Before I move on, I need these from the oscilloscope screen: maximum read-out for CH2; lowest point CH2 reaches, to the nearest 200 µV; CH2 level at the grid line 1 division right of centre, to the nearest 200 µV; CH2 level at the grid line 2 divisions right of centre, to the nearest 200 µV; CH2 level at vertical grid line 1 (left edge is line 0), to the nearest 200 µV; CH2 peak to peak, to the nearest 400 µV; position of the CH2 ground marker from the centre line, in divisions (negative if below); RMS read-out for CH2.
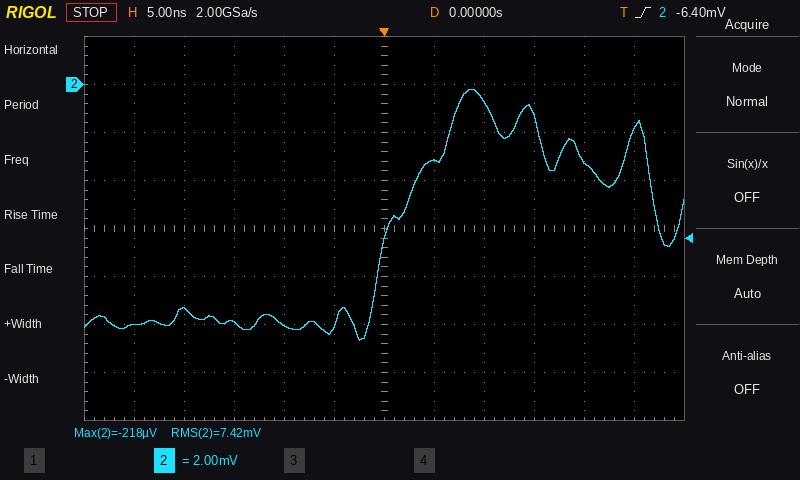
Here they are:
-218 µV
-10.6 mV
-3.2 mV
-800 µV
-10.0 mV
10.4 mV
+3.0 div
7.42 mV
